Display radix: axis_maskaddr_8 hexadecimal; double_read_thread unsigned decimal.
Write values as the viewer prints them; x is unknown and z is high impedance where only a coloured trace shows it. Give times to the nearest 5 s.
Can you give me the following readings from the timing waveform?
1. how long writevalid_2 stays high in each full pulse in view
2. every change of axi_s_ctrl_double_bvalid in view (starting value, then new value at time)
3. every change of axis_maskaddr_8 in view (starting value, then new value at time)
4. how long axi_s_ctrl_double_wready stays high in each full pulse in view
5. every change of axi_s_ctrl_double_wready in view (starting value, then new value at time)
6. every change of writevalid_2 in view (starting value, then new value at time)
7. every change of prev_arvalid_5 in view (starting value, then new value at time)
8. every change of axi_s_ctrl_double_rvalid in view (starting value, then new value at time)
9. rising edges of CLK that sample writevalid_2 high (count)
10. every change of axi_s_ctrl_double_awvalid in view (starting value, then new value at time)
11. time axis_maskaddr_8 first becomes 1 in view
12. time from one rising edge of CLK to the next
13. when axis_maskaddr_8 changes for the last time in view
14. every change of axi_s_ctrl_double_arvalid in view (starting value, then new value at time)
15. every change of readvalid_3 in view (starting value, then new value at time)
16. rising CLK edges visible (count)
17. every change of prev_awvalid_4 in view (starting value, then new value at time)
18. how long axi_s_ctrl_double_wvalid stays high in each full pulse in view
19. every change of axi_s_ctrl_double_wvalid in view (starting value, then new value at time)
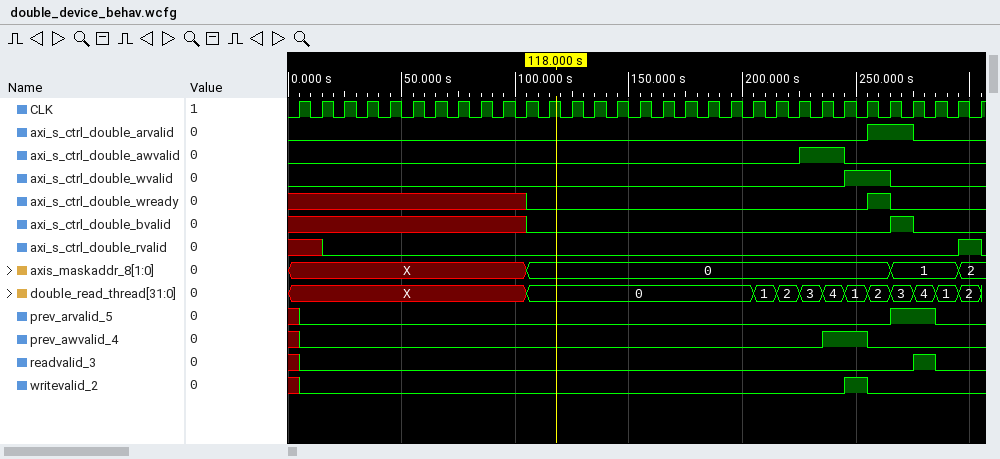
10 s
x, 0 at 105 s, 1 at 265 s, 0 at 275 s
X, 0 at 105 s, 1 at 265 s, 2 at 295 s
10 s
x, 0 at 105 s, 1 at 255 s, 0 at 265 s
x, 0 at 5 s, 1 at 245 s, 0 at 255 s
x, 0 at 5 s, 1 at 265 s, 0 at 285 s
x, 0 at 15 s, 1 at 295 s, 0 at 305 s
1
0, 1 at 225 s, 0 at 245 s
265 s
10 s
295 s
0, 1 at 255 s, 0 at 275 s
x, 0 at 5 s, 1 at 275 s, 0 at 285 s
31
x, 0 at 5 s, 1 at 235 s, 0 at 255 s
20 s
0, 1 at 245 s, 0 at 265 s
